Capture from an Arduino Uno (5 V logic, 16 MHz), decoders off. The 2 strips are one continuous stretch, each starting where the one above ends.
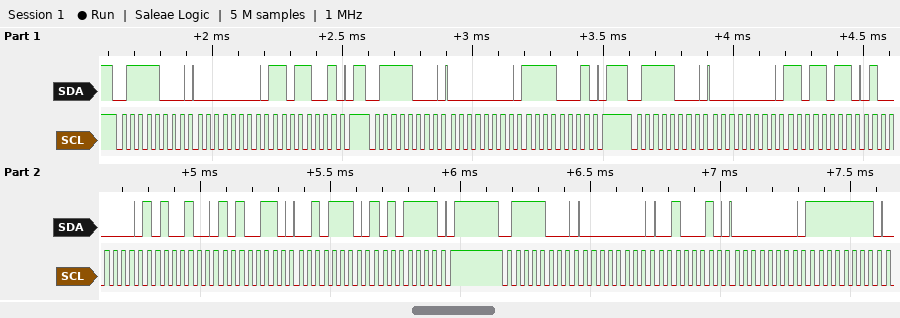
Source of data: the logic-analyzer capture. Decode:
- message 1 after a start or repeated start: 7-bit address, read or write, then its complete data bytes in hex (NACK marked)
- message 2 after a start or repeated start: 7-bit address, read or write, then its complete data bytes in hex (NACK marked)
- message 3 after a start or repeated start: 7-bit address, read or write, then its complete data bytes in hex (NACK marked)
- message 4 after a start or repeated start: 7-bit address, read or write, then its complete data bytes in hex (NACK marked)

0x3C write: 00 D9
0x3C write: 00 F1
0x3C write: 00 DB 40 A4 A6 2E AF
0x3C write: 00 22 00 FF
